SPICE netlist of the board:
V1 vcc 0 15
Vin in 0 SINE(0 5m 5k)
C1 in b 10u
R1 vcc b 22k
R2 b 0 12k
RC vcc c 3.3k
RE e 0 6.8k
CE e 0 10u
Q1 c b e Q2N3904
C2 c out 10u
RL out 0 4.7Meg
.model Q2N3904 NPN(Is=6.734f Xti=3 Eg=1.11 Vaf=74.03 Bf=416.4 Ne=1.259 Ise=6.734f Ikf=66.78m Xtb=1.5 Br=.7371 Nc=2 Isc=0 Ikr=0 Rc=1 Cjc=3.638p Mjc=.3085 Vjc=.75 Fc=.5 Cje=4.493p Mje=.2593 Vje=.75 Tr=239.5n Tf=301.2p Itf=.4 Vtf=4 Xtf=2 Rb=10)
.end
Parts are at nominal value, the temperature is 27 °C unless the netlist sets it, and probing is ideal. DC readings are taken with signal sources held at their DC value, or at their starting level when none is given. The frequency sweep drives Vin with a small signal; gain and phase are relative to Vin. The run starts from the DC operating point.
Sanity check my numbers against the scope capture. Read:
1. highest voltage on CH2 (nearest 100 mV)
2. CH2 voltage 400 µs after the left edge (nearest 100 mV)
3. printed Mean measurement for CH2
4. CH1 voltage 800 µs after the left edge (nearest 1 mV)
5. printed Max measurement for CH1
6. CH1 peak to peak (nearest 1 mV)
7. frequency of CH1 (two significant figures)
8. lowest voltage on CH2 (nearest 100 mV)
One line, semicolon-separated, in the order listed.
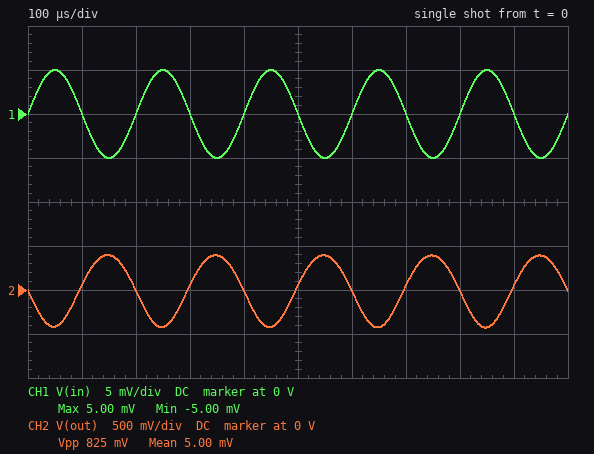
400 mV; 0 V; 5.00 mV; 0 V; 5.00 mV; 10 mV; 5.0 kHz; -400 mV
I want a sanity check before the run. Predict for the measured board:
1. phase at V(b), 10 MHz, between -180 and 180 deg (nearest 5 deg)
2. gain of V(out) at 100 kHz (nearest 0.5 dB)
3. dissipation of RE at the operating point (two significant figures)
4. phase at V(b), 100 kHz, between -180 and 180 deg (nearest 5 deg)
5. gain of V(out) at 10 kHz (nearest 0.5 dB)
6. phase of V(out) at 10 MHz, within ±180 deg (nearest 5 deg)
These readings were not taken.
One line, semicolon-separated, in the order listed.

0 deg; 38.5 dB; 3.1 mW; 0 deg; 38.5 dB; 155 deg
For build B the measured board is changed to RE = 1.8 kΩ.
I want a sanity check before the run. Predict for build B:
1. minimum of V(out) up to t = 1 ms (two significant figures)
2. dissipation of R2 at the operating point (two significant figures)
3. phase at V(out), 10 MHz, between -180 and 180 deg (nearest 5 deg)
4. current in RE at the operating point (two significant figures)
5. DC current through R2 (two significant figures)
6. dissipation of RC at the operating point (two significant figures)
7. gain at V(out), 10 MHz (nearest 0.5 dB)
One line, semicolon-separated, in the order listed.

-1.4 V; 2.2 mW; 135 deg; 2.5 mA; 430 µA; 20 mW; 46.0 dB
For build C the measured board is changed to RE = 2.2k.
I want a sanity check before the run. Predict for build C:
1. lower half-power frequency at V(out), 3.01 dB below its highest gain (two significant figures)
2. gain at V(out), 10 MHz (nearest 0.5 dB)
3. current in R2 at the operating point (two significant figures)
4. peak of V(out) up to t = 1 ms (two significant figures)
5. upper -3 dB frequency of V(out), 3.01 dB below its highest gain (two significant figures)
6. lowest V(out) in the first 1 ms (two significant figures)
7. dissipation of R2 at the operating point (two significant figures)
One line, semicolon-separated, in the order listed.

1.1 kHz; 45.5 dB; 430 µA; 1.1 V; 13 MHz; -1.2 V; 2.2 mW
